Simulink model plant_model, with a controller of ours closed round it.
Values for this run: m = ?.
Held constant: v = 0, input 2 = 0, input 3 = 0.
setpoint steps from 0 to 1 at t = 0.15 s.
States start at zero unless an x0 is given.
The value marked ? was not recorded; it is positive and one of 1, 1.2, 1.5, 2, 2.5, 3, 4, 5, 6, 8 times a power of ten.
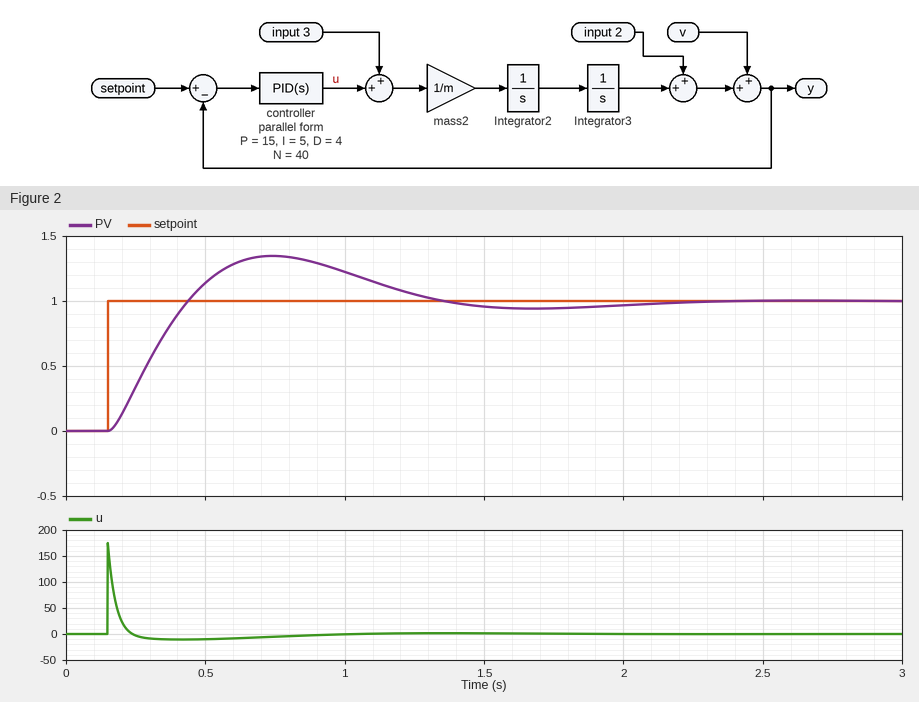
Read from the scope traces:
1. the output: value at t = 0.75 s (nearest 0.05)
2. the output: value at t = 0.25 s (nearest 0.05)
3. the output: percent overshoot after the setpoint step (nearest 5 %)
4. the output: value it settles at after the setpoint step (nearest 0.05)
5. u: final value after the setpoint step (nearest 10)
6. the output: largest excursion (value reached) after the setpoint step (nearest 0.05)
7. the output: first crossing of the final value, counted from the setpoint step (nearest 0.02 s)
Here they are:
1.35
0.35
35 %
1.00
0
1.35
0.28 s
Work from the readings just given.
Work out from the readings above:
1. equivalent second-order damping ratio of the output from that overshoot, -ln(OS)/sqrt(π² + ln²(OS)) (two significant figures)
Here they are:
0.32
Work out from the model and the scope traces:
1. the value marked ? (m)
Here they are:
1
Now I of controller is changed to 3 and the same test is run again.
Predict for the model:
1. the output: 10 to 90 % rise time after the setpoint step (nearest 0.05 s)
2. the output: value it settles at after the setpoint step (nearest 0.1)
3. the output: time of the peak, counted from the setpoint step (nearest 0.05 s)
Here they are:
0.20 s
1.0
0.60 s
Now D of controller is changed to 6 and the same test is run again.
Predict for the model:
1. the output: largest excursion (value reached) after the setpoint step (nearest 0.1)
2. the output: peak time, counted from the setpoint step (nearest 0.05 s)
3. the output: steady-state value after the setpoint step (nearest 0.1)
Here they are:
1.2
0.50 s
1.0
